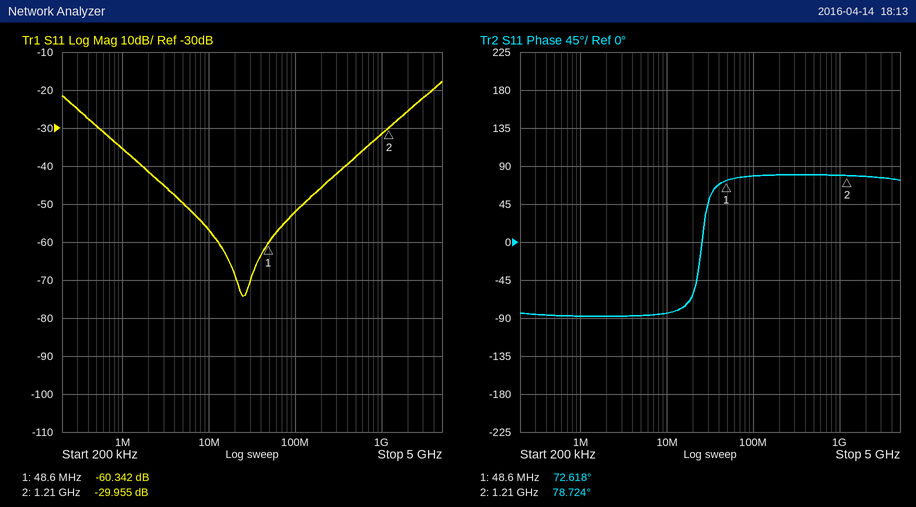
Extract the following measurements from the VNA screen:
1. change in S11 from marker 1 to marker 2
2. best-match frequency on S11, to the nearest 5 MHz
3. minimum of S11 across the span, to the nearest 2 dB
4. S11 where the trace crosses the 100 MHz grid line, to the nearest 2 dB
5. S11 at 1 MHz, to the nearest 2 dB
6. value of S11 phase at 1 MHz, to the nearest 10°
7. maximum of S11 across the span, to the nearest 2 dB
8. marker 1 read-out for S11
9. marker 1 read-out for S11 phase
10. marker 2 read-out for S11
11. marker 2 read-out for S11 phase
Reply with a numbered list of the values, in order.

1. 30.387 dB
2. 25 MHz
3. -74 dB
4. -52 dB
5. -36 dB
6. -90°
7. -18 dB
8. -60.342 dB
9. 72.618°
10. -29.955 dB
11. 78.724°
